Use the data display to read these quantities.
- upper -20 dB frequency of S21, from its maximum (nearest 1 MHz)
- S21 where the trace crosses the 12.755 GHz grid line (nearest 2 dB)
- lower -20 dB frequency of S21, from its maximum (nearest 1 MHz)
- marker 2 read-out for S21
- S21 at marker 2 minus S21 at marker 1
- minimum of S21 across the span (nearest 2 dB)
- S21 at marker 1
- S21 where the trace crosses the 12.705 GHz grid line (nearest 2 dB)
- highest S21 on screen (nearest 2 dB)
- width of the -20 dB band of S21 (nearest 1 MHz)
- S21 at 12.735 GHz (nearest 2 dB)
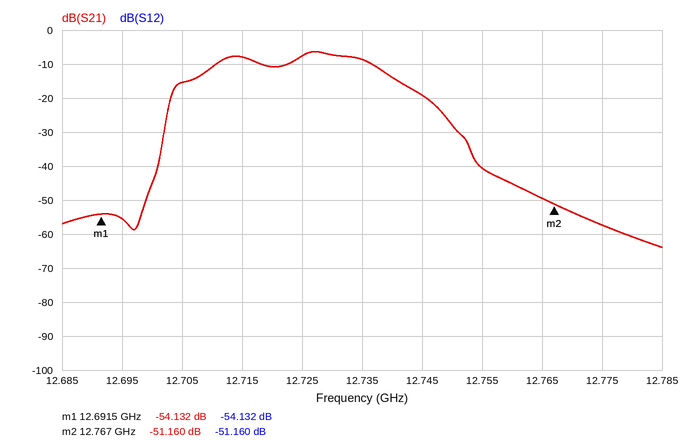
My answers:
12.749 GHz
-40 dB
12.702 GHz
-51.160 dB
2.972 dB
-64 dB
-54.132 dB
-16 dB
-6 dB
47 MHz
-8 dB
